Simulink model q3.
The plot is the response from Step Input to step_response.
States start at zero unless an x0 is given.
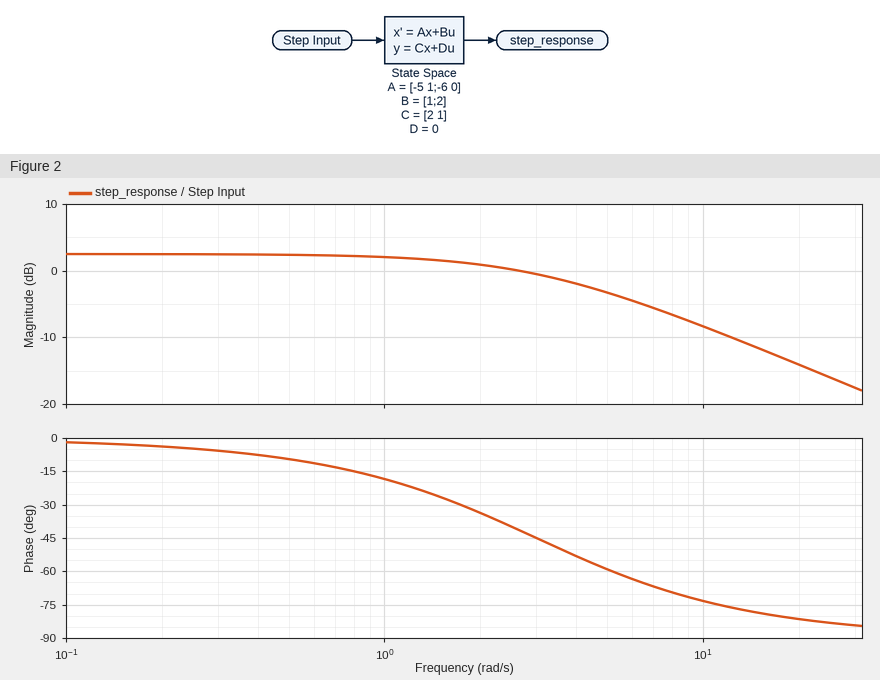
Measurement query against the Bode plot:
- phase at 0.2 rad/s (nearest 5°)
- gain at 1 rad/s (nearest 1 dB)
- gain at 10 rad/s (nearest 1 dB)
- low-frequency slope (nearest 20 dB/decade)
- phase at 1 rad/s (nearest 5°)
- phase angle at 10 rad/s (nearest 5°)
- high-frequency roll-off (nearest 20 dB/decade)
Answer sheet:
-5°
2 dB
-8 dB
0 dB/decade
-20°
-75°
-20 dB/decade
